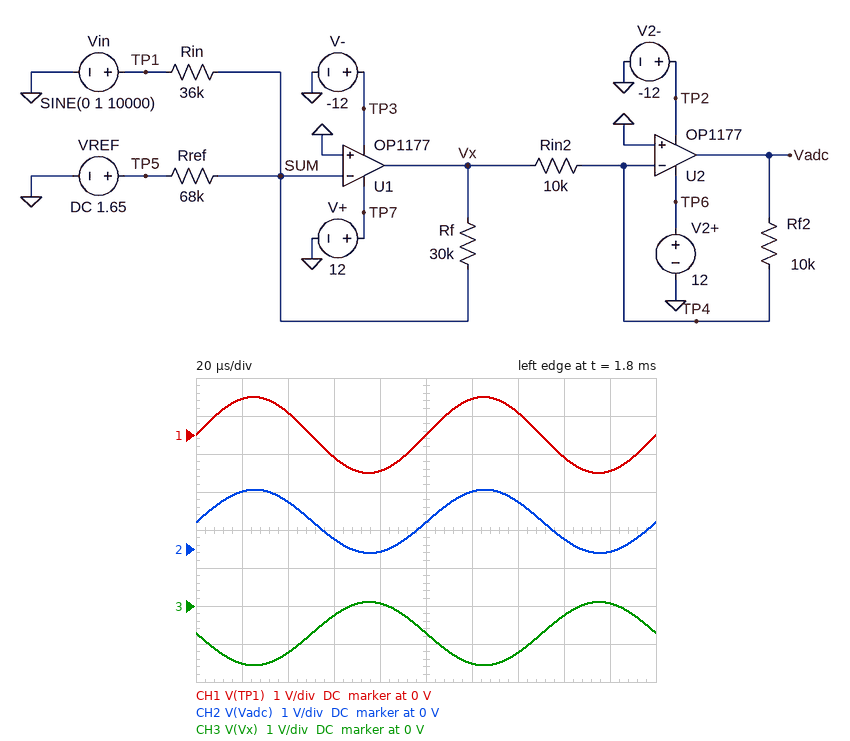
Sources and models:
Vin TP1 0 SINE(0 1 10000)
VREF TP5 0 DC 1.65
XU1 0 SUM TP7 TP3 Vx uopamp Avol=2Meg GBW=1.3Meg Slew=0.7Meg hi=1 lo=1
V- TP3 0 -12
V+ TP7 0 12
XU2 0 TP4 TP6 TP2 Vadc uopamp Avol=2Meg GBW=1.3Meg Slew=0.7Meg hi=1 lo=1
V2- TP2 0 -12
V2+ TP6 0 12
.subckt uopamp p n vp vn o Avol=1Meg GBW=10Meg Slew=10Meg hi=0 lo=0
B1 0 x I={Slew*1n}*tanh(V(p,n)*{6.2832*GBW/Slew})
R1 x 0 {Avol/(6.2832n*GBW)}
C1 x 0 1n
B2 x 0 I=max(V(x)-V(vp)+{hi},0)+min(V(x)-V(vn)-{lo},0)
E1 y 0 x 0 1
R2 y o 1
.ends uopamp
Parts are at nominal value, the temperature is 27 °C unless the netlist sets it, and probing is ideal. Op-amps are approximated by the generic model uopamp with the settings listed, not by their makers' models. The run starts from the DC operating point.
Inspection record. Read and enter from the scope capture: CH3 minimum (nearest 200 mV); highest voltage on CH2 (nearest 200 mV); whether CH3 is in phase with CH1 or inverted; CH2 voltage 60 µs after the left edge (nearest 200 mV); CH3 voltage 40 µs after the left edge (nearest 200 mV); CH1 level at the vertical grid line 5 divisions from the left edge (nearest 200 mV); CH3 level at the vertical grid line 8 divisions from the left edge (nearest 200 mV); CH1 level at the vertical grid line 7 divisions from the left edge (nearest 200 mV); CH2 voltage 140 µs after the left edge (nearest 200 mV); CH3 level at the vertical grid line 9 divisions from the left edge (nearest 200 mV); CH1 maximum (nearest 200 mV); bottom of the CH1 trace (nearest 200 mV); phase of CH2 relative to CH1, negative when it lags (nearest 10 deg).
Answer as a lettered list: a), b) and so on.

a) -1.6 V
b) 1.6 V
c) inverted
d) 200 mV
e) -1.2 V
f) 0 V
g) -200 mV
h) 600 mV
i) 1.2 V
j) 0 V
k) 1.0 V
l) -1.0 V
m) 0 deg
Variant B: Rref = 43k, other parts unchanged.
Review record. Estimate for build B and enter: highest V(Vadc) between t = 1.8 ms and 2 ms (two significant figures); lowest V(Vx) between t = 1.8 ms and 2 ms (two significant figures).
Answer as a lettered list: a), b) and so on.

a) 2.0 V
b) -2.0 V
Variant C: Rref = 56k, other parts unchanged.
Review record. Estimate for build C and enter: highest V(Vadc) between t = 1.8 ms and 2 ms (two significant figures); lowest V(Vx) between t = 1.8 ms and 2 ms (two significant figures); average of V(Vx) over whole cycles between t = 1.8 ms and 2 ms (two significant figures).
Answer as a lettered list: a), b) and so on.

a) 1.7 V
b) -1.7 V
c) -880 mV
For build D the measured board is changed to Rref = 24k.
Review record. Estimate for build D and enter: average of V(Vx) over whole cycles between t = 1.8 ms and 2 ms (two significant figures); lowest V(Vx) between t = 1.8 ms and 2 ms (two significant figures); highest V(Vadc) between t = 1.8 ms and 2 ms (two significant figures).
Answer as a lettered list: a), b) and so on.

a) -2.1 V
b) -2.9 V
c) 2.9 V
